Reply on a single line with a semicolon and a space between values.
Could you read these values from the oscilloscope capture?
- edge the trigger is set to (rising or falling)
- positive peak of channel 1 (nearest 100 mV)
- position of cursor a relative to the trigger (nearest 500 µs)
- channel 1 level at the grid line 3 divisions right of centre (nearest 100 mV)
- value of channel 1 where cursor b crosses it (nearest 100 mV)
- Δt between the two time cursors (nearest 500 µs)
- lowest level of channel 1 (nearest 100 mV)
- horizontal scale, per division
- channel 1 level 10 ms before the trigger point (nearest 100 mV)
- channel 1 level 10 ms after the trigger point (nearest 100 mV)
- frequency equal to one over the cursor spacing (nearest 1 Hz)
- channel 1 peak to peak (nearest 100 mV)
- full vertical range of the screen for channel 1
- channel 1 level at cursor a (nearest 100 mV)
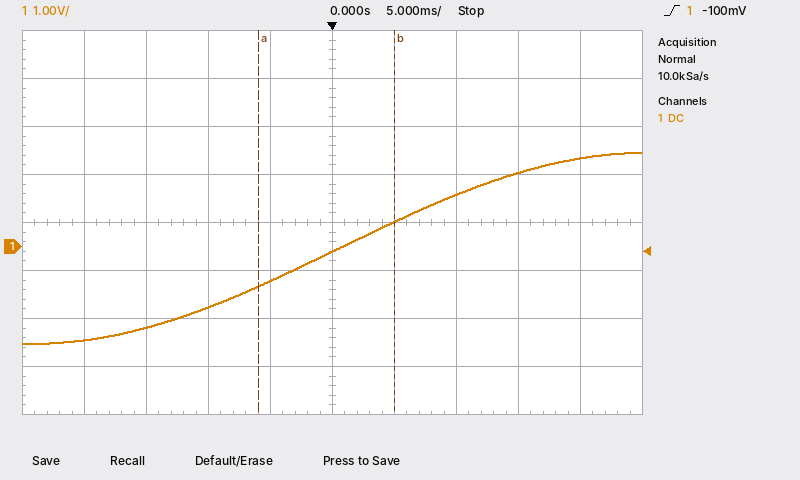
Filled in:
rising; 2.0 V; -6.0 ms; 1.5 V; 500 mV; 11.0 ms; -2.0 V; 5 ms; -1.3 V; 1.1 V; 91 Hz; 4.0 V; 8 V; -800 mV
